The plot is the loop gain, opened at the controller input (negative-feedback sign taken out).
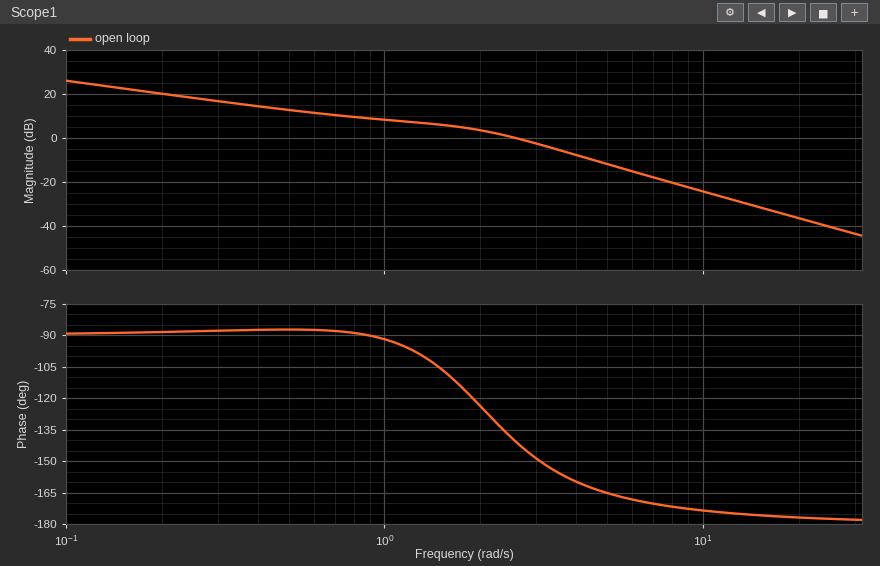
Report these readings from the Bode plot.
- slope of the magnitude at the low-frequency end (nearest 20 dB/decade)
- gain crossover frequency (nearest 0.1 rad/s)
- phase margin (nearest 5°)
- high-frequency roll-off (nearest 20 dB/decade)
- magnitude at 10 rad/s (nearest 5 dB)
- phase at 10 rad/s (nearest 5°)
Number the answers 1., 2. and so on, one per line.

1. -20 dB/decade
2. 2.6 rad/s
3. 40°
4. -40 dB/decade
5. -25 dB
6. -175°
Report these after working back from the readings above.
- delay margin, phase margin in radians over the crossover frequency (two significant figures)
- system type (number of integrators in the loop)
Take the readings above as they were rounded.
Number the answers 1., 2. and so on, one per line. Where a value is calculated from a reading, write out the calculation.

1. 40 × π / 180 / 2.6 = 0.27 s
2. 1
